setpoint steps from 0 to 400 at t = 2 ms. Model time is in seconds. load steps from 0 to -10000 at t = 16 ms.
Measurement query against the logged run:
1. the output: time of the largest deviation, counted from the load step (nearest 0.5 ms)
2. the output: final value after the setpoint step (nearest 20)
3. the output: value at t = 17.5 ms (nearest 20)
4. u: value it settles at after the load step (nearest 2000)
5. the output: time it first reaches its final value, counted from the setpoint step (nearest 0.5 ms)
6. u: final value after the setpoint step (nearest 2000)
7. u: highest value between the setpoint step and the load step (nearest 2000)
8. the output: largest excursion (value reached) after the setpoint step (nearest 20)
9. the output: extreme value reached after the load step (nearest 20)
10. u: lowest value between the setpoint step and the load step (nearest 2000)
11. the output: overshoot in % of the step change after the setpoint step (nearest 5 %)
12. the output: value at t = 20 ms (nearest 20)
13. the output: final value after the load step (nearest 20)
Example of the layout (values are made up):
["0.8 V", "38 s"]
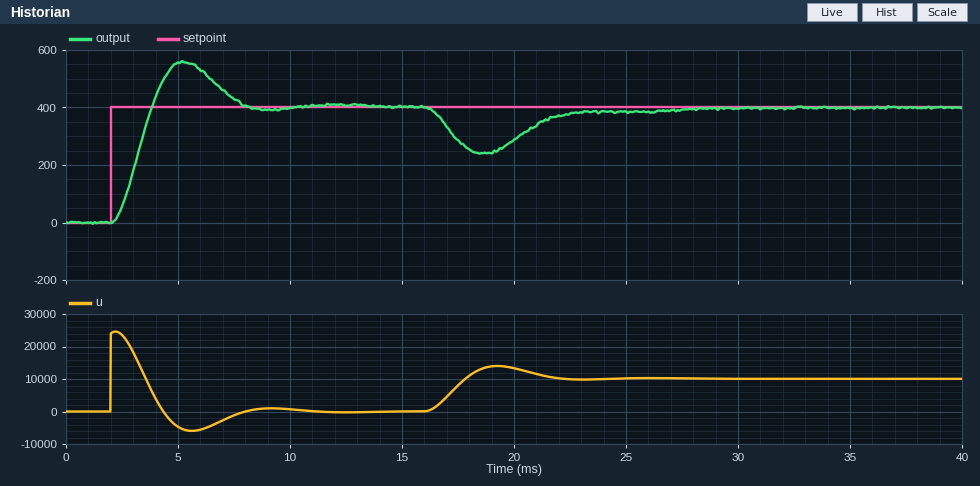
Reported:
["2.5 ms", "400", "280", "10000", "2.0 ms", "0", "24000", "560", "240", "-6000", "40 %", "280", "400"]
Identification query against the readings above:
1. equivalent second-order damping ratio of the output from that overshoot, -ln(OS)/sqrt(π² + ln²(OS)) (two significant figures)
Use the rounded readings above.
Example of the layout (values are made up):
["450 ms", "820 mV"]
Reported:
["0.28"]
